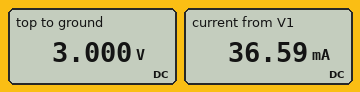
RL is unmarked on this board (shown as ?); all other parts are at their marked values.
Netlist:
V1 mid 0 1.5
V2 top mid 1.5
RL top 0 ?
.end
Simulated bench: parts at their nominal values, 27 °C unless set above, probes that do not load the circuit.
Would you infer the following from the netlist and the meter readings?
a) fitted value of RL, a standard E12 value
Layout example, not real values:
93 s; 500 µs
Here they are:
82 Ω
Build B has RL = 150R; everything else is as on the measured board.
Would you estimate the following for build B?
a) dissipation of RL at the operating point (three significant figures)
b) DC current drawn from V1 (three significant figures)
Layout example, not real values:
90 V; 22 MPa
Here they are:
60.0 mW; 20.0 mA
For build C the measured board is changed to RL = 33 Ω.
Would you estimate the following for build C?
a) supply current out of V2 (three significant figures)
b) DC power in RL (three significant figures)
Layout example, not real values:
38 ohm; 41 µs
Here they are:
90.9 mA; 273 mW
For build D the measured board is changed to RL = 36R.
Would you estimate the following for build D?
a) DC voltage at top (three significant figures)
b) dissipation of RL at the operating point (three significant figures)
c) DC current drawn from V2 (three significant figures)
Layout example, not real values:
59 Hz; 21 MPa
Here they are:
3.00 V; 250 mW; 83.3 mA
